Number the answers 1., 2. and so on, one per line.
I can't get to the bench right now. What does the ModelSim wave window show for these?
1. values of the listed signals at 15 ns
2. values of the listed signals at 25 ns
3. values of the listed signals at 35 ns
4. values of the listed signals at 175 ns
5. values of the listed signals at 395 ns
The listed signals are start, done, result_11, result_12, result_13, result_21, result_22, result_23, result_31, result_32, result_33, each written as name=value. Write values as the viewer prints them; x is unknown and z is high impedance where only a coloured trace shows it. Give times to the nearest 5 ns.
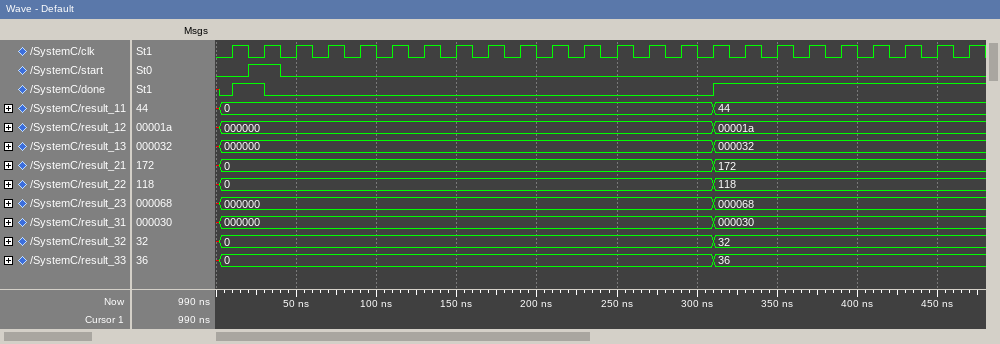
1. start=0, done=1, result_11=0, result_12=000000, result_13=000000, result_21=0, result_22=0, result_23=000000, result_31=000000, result_32=0, result_33=0
2. start=1, done=1, result_11=0, result_12=000000, result_13=000000, result_21=0, result_22=0, result_23=000000, result_31=000000, result_32=0, result_33=0
3. start=1, done=0, result_11=0, result_12=000000, result_13=000000, result_21=0, result_22=0, result_23=000000, result_31=000000, result_32=0, result_33=0
4. start=0, done=0, result_11=0, result_12=000000, result_13=000000, result_21=0, result_22=0, result_23=000000, result_31=000000, result_32=0, result_33=0
5. start=0, done=1, result_11=44, result_12=00001a, result_13=000032, result_21=172, result_22=118, result_23=000068, result_31=000030, result_32=32, result_33=36
